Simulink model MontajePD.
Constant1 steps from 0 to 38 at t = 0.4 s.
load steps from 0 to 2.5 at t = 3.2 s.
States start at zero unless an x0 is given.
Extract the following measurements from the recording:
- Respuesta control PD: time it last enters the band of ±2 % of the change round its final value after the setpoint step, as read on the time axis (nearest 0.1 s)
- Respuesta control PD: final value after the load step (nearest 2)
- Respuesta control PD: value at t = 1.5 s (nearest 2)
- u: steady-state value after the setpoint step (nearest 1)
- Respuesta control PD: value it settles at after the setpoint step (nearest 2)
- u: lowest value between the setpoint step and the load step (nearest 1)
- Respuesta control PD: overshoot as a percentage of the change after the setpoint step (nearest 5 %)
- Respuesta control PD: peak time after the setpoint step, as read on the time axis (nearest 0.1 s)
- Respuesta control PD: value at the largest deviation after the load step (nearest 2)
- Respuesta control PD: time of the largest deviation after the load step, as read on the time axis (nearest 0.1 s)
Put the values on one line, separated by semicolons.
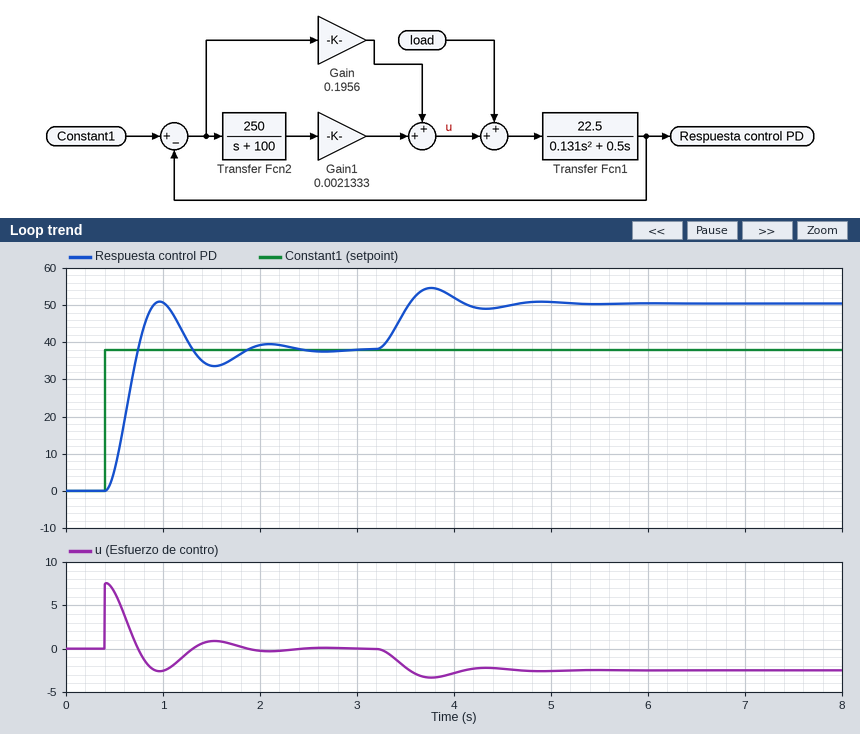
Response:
2.3 s; 50; 34; 0; 38; -3; 35 %; 1.0 s; 54; 3.8 s
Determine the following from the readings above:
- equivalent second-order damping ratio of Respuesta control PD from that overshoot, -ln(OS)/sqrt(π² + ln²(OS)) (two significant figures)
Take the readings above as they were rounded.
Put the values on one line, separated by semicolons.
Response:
0.32
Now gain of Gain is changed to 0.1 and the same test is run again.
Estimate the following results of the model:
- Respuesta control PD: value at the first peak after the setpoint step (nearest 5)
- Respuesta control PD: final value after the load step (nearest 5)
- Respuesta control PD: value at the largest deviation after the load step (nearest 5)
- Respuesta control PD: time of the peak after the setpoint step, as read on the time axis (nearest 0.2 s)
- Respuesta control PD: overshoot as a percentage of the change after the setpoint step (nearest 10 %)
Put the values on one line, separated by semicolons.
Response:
45; 60; 65; 1.2 s; 20 %
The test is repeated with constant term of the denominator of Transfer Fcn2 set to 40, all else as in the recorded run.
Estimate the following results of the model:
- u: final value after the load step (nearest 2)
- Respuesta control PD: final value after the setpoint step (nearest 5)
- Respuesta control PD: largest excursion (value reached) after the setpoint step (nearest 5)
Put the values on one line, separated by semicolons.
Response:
-2; 40; 50
